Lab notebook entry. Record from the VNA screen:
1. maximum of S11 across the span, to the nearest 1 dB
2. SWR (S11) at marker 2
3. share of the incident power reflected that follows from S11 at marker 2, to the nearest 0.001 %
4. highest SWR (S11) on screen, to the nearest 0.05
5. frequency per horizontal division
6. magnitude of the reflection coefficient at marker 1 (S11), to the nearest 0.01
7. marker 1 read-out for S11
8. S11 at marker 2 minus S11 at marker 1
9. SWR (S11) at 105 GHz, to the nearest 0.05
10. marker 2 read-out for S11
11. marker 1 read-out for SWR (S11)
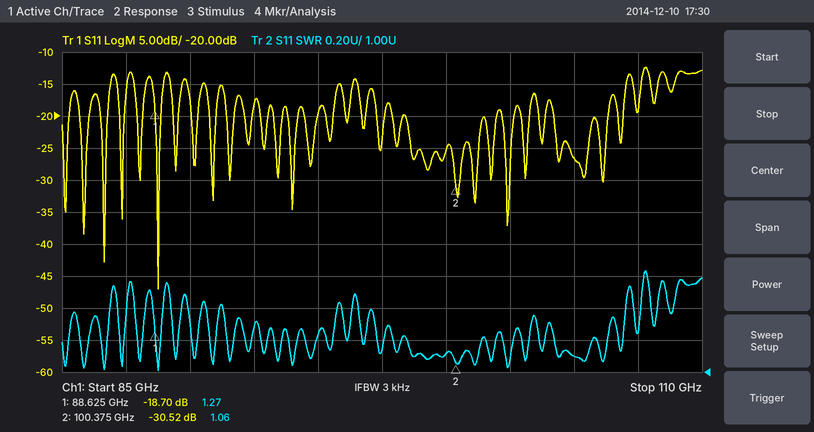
-12 dB
1.06
0.089 %
1.65
2.5 GHz
0.12
-18.70 dB
-11.82 dB
1.10
-30.52 dB
1.27
